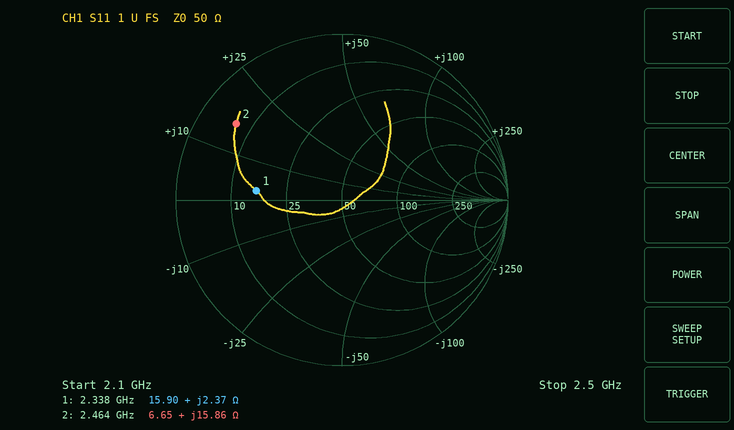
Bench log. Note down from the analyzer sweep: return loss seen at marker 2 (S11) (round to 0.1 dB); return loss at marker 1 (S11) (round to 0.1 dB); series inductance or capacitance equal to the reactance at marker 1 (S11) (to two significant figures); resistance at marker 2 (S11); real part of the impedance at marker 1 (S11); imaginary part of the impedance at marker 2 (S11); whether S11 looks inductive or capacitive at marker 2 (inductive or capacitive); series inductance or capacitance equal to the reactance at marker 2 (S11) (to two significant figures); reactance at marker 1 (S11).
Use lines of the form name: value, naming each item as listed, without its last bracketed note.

return loss seen at marker 2 (S11): 2.1 dB
return loss at marker 1 (S11): 5.7 dB
series inductance or capacitance equal to the reactance at marker 1 (S11): 160 pH
resistance at marker 2: 6.65 Ω
real part of the impedance at marker 1: 15.90 Ω
imaginary part of the impedance at marker 2: +15.86 Ω
whether S11 looks inductive or capacitive at marker 2: inductive
series inductance or capacitance equal to the reactance at marker 2 (S11): 1.0 nH
reactance at marker 1: +2.37 Ω
